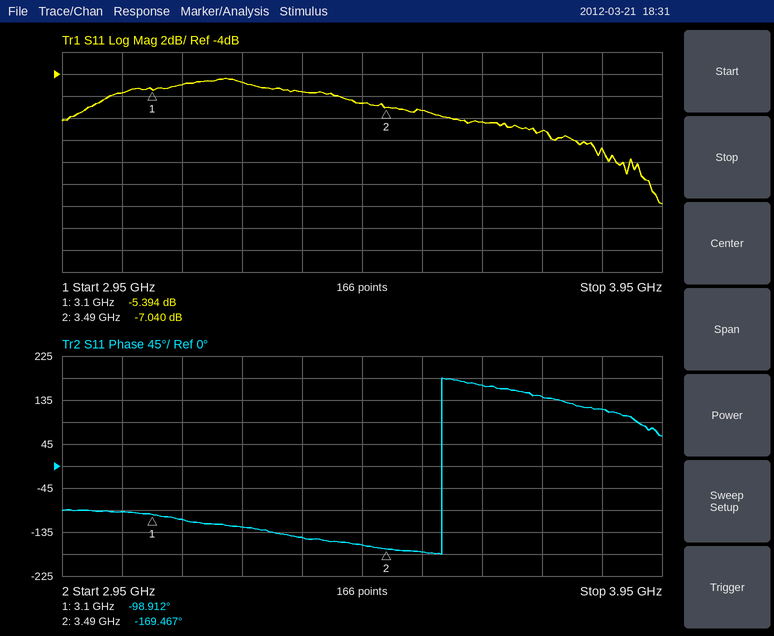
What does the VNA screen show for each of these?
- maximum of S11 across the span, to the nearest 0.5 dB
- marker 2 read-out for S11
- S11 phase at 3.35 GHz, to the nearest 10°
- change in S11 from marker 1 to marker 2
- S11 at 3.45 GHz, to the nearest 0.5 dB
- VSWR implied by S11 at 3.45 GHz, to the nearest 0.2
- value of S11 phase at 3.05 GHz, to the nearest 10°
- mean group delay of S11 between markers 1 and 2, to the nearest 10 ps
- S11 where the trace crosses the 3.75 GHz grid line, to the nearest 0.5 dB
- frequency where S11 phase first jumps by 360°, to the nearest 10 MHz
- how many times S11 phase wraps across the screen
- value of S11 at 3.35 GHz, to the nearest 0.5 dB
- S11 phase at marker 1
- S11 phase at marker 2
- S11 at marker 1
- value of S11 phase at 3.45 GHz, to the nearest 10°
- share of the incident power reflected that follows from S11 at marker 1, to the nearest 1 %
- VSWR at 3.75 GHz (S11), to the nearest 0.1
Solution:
-4.5 dB
-7.040 dB
-150°
-1.646 dB
-6.5 dB
2.8
-90°
500 ps
-9.0 dB
3.58 GHz
1
-5.5 dB
-98.912°
-169.467°
-5.394 dB
-160°
29 %
2.1
